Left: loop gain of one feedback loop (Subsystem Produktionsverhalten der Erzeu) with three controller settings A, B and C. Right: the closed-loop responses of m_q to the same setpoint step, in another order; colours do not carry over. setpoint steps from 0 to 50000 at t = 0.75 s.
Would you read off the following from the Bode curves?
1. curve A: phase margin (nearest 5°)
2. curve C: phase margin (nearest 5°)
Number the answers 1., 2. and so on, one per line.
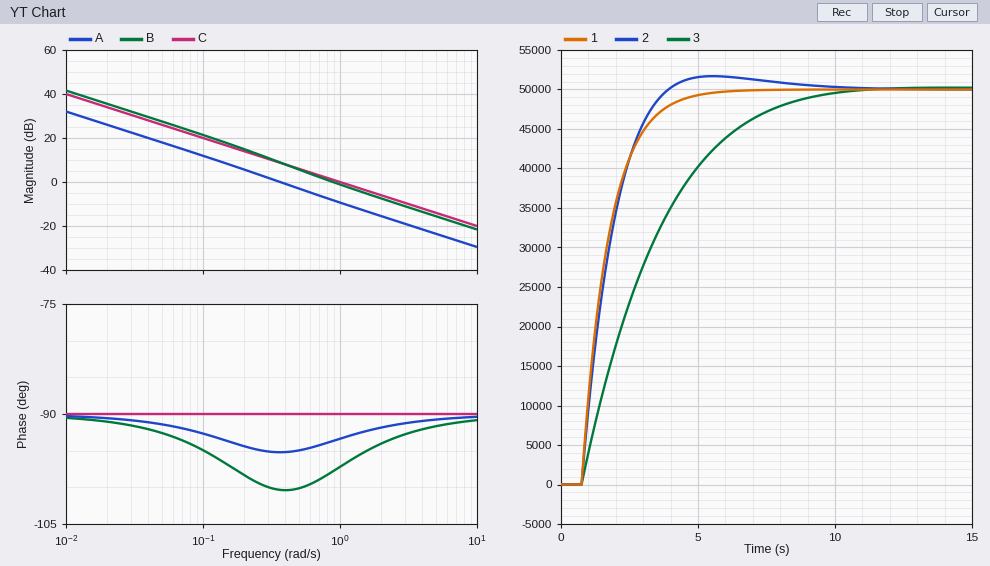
1. 85°
2. 90°
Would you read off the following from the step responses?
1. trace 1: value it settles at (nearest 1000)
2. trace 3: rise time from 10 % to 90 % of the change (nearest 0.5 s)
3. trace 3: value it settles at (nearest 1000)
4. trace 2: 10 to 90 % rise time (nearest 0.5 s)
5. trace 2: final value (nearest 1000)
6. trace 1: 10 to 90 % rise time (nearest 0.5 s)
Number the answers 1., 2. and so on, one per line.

1. 50000
2. 5.5 s
3. 50000
4. 2.0 s
5. 50000
6. 2.0 s
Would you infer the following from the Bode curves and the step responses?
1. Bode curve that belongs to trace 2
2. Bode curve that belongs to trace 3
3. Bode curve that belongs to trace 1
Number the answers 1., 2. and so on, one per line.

1. B
2. A
3. C
